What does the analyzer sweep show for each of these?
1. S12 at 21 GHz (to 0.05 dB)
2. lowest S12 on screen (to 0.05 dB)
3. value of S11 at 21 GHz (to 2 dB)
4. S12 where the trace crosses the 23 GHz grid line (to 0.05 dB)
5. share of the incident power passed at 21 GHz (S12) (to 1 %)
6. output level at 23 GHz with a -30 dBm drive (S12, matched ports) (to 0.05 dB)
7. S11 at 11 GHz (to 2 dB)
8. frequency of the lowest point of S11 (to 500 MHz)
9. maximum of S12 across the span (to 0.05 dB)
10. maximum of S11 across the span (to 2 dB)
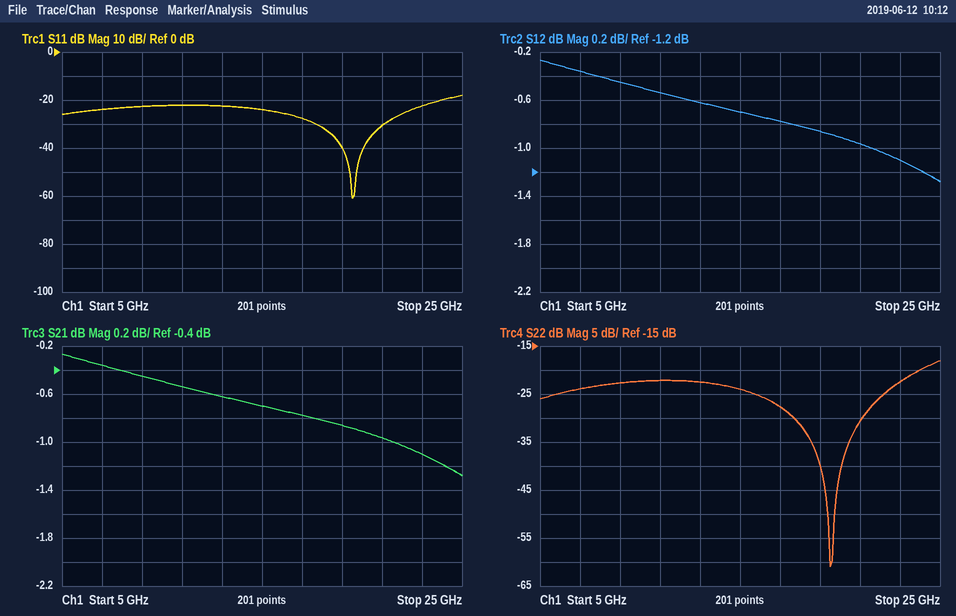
-0.95 dB
-1.30 dB
-30 dB
-1.10 dB
80 %
-31.10 dBm
-22 dB
19.5 GHz
-0.25 dB
-18 dB
